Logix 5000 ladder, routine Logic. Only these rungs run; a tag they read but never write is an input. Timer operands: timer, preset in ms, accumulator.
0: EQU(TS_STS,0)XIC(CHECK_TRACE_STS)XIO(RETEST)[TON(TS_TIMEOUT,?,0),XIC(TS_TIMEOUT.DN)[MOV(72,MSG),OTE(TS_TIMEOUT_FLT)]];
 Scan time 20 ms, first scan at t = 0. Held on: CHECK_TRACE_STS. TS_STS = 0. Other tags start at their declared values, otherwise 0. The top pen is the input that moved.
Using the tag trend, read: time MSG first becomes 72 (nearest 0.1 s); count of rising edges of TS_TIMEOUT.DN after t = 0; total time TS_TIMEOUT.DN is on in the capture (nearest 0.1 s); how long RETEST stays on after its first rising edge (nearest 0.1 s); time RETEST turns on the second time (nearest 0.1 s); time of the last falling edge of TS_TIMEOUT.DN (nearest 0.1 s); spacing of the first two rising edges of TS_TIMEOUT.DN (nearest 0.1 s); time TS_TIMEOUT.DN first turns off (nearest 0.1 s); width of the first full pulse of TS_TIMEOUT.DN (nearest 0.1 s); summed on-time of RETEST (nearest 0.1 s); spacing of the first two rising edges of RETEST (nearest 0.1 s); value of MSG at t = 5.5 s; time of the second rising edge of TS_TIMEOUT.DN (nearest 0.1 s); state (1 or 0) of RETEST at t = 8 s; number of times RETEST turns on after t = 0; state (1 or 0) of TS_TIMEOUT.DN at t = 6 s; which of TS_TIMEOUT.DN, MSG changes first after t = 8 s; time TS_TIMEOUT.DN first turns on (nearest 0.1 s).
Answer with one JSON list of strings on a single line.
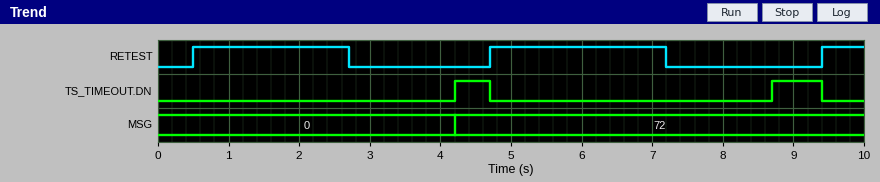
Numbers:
["4.2 s", "2", "1.2 s", "2.2 s", "4.7 s", "9.4 s", "4.5 s", "4.7 s", "0.5 s", "5.3 s", "4.2 s", "72", "8.7 s", "0", "3", "0", "TS_TIMEOUT.DN", "4.2 s"]
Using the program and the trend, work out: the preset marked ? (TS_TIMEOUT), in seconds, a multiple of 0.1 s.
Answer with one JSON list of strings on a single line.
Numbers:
["1.5 s"]
